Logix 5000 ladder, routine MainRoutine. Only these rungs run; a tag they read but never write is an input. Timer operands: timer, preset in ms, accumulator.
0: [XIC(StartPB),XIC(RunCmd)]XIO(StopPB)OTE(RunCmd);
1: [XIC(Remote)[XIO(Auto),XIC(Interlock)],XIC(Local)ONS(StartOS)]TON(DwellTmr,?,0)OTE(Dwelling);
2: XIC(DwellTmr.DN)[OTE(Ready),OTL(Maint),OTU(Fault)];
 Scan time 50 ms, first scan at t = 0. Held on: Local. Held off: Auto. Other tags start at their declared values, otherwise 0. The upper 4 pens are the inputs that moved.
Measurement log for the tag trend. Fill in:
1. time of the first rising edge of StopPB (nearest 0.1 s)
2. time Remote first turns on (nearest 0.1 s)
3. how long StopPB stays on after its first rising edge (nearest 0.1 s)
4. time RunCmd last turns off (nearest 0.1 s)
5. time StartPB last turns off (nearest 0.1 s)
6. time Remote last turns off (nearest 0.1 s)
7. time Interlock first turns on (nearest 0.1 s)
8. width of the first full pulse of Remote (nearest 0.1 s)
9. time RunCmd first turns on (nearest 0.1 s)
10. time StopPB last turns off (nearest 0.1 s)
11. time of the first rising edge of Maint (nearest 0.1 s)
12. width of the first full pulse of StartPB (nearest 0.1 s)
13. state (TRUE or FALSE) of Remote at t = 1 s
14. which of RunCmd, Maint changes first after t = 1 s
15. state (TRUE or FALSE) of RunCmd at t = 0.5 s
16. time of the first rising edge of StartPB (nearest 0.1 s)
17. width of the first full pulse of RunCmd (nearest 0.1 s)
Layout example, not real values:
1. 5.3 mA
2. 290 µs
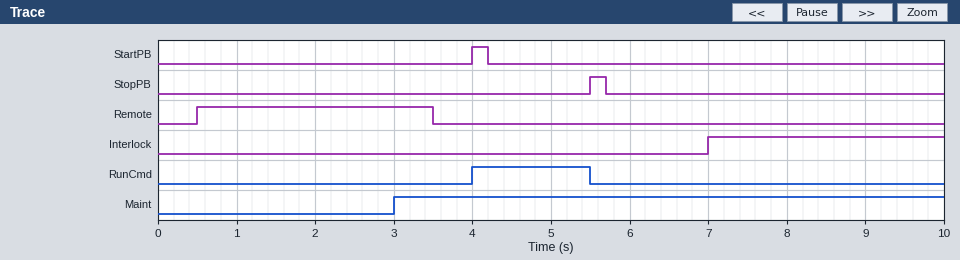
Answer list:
1. 5.5 s
2. 0.5 s
3. 0.2 s
4. 5.5 s
5. 4.2 s
6. 3.5 s
7. 7.0 s
8. 3.0 s
9. 4.0 s
10. 5.7 s
11. 3.0 s
12. 0.2 s
13. TRUE
14. Maint
15. FALSE
16. 4.0 s
17. 1.5 s
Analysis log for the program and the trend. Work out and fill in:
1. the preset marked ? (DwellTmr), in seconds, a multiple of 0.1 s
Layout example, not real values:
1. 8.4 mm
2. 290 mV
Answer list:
1. 2.5 s
